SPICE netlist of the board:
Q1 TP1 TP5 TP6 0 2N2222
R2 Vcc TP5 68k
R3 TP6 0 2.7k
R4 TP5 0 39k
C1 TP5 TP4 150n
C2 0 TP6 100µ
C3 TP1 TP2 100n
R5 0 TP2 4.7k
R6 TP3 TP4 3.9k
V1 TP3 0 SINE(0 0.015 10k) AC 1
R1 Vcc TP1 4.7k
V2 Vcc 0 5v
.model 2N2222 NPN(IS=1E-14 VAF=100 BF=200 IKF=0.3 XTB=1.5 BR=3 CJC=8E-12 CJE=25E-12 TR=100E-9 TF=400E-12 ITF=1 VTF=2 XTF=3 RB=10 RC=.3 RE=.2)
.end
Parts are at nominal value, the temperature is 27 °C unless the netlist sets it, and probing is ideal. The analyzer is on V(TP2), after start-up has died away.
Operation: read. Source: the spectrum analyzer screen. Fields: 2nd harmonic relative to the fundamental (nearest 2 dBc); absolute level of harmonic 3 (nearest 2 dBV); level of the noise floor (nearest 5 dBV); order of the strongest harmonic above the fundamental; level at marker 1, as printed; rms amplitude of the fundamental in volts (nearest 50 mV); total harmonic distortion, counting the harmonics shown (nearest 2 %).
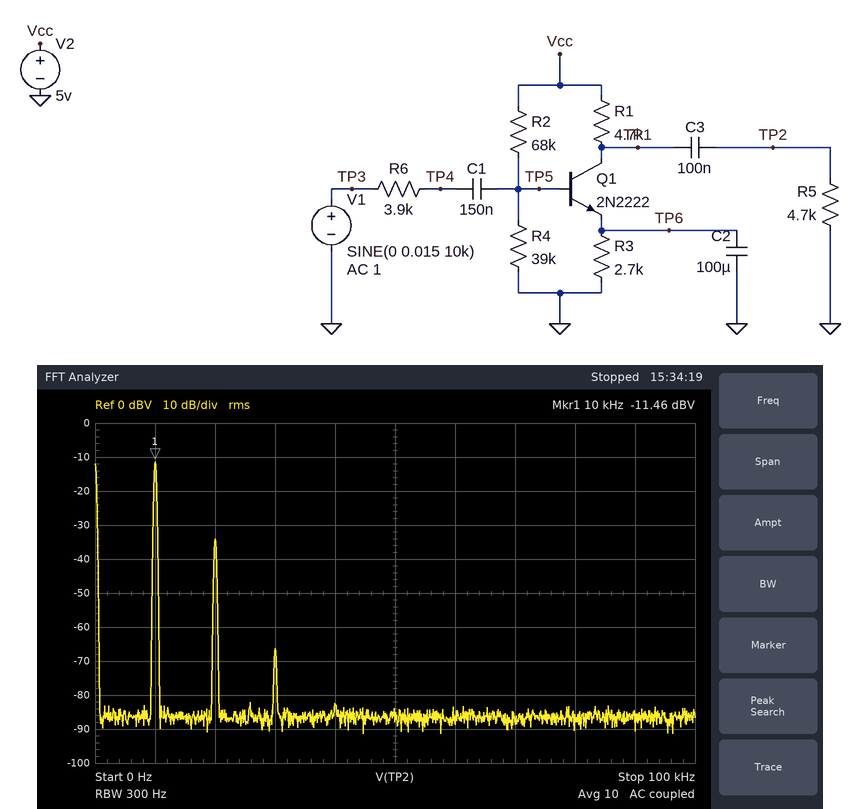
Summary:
-22 dBc
-66 dBV
-85 dBV
2
-11.46 dBV
250 mV
8 %
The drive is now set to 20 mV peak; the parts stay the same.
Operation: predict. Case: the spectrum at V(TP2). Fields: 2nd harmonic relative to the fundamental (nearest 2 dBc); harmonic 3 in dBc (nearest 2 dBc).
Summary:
-20 dBc
-50 dBc
